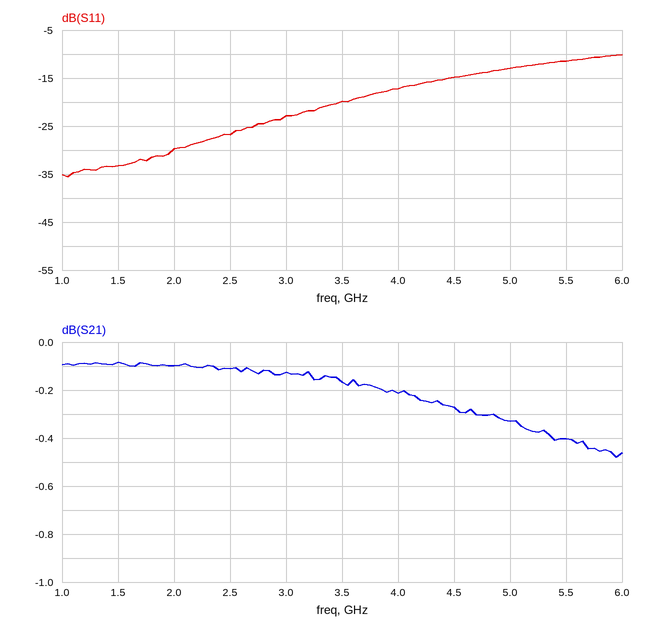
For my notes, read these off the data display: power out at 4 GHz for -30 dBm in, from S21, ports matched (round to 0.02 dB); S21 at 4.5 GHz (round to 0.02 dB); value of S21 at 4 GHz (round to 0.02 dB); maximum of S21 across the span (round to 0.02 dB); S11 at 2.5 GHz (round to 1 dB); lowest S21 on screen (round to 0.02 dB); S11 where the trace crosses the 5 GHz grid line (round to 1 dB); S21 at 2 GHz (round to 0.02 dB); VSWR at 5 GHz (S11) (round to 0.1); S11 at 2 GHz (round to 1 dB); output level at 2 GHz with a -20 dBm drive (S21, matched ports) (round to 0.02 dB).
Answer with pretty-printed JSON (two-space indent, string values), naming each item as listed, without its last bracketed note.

{
  "power out at 4 GHz for -30 dBm in, from S21, ports matched": "-30.22 dBm",
  "S21 at 4.5 GHz": "-0.28 dB",
  "value of S21 at 4 GHz": "-0.22 dB",
  "maximum of S21 across the span": "-0.08 dB",
  "S11 at 2.5 GHz": "-27 dB",
  "lowest S21 on screen": "-0.48 dB",
  "S11 where the trace crosses the 5 GHz grid line": "-13 dB",
  "S21 at 2 GHz": "-0.10 dB",
  "VSWR at 5 GHz (S11)": "1.6",
  "S11 at 2 GHz": "-30 dB",
  "output level at 2 GHz with a -20 dBm drive (S21, matched ports)": "-20.10 dBm"
}
